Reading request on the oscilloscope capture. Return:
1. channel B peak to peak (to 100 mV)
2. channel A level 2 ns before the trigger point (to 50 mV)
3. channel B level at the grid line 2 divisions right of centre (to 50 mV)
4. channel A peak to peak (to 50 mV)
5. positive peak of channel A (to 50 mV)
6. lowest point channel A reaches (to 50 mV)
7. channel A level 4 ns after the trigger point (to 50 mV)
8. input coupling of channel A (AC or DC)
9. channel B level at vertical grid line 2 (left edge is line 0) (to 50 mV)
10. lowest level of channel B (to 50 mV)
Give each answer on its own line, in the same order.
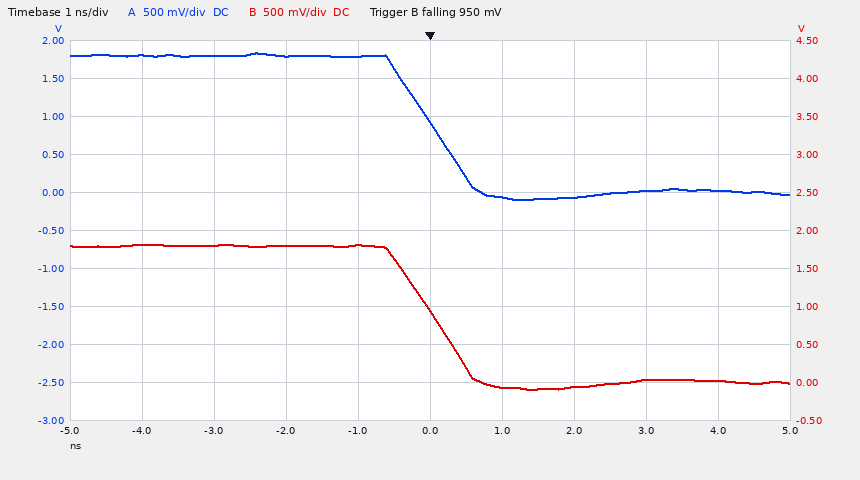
1.90 V
1.80 V
-50 mV
1.95 V
1.85 V
-100 mV
50 mV
DC
1.80 V
-100 mV
